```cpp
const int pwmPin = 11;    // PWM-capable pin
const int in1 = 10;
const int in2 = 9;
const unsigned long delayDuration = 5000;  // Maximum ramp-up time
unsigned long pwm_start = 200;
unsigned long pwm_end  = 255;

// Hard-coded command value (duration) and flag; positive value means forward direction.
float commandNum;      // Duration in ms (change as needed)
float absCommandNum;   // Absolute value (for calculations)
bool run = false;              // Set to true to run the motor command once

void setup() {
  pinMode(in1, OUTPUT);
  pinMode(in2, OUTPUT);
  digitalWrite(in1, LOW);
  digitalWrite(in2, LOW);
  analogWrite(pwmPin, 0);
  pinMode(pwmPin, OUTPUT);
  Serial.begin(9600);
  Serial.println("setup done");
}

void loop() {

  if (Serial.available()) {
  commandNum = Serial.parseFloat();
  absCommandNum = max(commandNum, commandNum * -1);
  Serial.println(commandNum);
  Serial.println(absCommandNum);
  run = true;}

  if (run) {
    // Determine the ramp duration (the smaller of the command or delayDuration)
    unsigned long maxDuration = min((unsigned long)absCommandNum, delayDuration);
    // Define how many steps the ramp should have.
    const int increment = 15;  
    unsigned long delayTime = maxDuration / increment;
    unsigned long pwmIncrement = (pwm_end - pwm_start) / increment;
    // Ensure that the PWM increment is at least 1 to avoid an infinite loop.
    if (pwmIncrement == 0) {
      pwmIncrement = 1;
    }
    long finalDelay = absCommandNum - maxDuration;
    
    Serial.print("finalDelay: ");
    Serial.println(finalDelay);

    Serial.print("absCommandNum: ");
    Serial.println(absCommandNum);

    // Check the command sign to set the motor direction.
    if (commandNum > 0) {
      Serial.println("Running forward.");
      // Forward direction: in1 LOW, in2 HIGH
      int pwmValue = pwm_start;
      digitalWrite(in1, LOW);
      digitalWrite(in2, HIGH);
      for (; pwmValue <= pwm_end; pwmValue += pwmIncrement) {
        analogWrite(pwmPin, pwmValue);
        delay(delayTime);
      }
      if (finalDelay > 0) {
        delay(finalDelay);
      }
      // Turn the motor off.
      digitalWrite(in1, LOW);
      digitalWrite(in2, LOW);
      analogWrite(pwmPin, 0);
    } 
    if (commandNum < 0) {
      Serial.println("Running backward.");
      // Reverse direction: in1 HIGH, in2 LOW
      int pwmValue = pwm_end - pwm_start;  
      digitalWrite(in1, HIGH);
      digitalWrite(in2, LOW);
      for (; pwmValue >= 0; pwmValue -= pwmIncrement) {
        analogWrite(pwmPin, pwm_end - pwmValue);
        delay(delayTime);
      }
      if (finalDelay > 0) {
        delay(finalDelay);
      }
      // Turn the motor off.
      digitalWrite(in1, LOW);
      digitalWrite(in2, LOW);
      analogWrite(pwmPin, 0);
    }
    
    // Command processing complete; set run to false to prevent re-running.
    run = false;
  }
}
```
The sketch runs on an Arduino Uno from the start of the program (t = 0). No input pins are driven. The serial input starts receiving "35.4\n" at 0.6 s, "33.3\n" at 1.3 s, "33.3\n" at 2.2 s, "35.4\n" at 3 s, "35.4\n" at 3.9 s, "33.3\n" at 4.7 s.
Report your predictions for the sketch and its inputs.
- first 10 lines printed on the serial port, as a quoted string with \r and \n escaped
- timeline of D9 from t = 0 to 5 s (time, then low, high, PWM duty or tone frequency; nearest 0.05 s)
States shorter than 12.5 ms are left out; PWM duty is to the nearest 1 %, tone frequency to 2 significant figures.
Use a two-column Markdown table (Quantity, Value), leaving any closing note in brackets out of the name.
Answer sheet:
| Quantity | Value |
|---|---|
| first 10 lines printed on the serial port, as a quoted string with \r and \n escaped | "setup done\r\n35.40\r\n35.40\r\nfinalDelay: 0\r\nabsCommandNum: 35.40\r\nRunning forward.\r\n33.30\r\n33.30\r\nfinalDelay: 0\r\nabsCommandNum: 33.30\r\n" |
| timeline of D9 from t = 0 to 5 s | 0 s low; 0.6 s high; 0.65 s low; 1.3 s high; 1.35 s low; 2.2 s high; 2.25 s low; 3 s high; 3.05 s low; 3.9 s high; 3.95 s low; 4.7 s high; 4.75 s low |
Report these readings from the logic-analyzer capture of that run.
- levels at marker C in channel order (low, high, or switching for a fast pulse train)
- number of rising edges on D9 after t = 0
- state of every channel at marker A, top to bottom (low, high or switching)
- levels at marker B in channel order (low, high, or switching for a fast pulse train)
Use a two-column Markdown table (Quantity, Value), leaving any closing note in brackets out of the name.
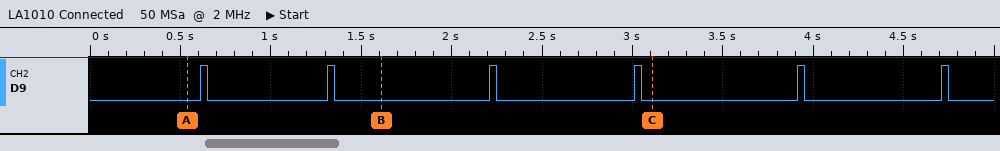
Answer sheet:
| Quantity | Value |
|---|---|
| levels at marker C in channel order | D9 low |
| number of rising edges on D9 after t = 0 | 6 |
| state of every channel at marker A, top to bottom | D9 low |
| levels at marker B in channel order | D9 low |
